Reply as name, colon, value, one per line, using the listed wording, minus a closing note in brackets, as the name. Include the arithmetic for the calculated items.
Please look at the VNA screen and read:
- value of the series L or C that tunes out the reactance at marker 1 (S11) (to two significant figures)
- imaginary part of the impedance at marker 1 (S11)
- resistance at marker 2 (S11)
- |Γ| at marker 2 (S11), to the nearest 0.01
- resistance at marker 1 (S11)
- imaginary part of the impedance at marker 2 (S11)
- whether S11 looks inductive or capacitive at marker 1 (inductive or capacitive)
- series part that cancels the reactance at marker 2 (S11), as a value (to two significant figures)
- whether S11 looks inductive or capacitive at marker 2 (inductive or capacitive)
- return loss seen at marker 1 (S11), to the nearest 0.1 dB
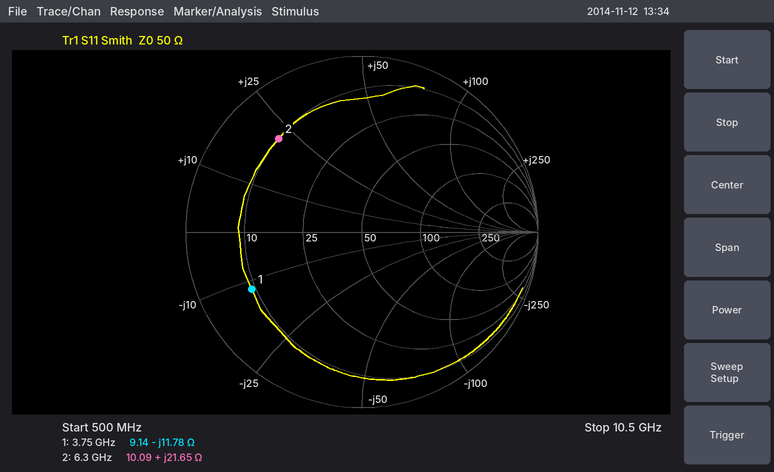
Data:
value of the series L or C that tunes out the reactance at marker 1 (S11): L = 11.78 Ω/(2π × 3.75 GHz) ≈ 500 pH
imaginary part of the impedance at marker 1: -11.78 Ω
resistance at marker 2: 10.09 Ω
|Γ| at marker 2 (S11), to the nearest 0.01: 0.71
resistance at marker 1: 9.14 Ω
imaginary part of the impedance at marker 2: +21.65 Ω
whether S11 looks inductive or capacitive at marker 1: capacitive
series part that cancels the reactance at marker 2 (S11), as a value: C = 1/(2π × 6.3 GHz × 21.65 Ω) ≈ 1.2 pF
whether S11 looks inductive or capacitive at marker 2: inductive
return loss seen at marker 1 (S11), to the nearest 0.1 dB: 3.0 dB
